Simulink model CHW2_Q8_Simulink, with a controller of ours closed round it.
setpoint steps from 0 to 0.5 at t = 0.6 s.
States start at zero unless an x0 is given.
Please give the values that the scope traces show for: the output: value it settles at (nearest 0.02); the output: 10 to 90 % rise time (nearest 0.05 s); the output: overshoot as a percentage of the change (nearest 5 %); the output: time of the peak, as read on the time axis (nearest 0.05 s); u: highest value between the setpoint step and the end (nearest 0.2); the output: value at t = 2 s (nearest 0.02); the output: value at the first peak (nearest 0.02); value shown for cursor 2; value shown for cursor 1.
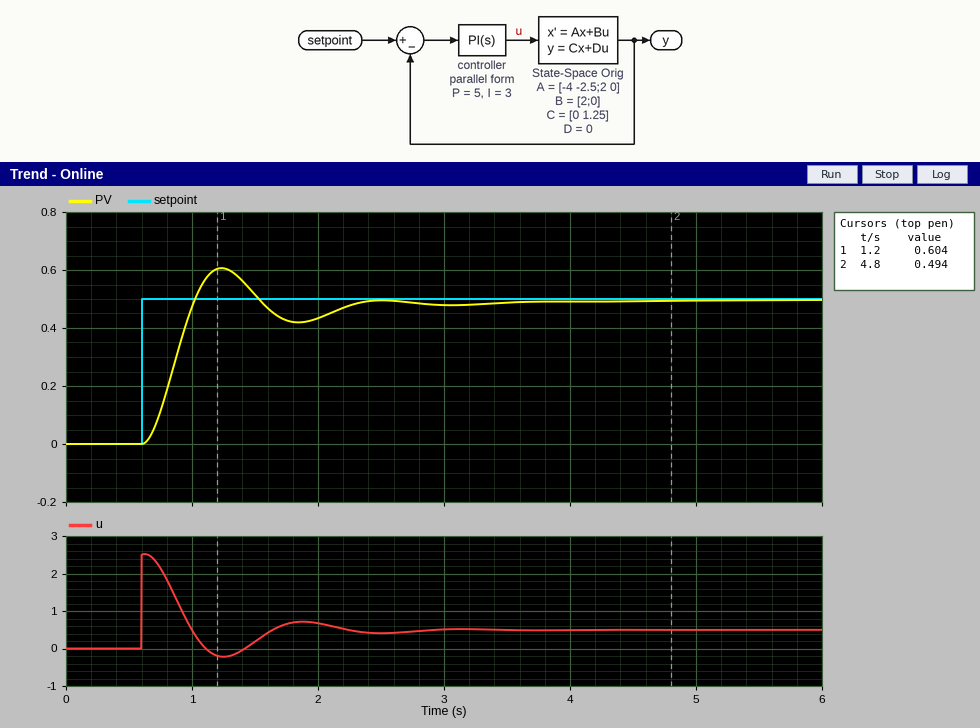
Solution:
0.50
0.30 s
20 %
1.25 s
2.6
0.44
0.60
0.494
0.604
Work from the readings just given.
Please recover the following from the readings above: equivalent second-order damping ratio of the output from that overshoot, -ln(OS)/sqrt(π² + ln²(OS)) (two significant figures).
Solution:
0.46
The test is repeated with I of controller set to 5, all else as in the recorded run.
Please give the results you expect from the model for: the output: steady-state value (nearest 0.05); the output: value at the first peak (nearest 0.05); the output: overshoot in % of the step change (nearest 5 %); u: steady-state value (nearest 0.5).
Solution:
0.50
0.65
30 %
0.5
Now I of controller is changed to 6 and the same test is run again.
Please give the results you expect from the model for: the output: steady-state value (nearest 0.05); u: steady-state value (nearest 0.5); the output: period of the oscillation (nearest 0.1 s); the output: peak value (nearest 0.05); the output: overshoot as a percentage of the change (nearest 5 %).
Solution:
0.50
0.5
1.3 s
0.65
35 %
